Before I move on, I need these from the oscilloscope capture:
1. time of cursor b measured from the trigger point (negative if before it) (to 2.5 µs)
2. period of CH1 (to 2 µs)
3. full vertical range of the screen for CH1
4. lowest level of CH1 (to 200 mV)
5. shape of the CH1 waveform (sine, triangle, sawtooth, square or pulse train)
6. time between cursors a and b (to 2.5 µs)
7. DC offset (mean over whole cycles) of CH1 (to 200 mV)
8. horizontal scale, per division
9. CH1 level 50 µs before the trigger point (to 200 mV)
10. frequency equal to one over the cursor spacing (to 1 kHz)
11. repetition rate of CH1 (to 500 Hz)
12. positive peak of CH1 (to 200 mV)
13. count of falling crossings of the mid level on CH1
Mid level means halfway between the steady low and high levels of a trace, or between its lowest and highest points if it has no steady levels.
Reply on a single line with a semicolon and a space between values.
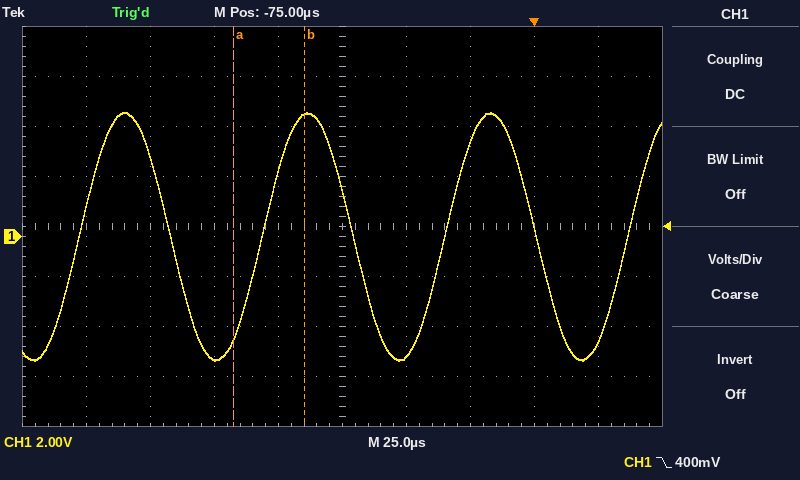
-90.0 µs; 72 µs; 16 V; -5.0 V; sine; 27.5 µs; 0.0 V; 25 µs; -4.8 V; 36 kHz; 14.0 kHz; 5.0 V; 3
